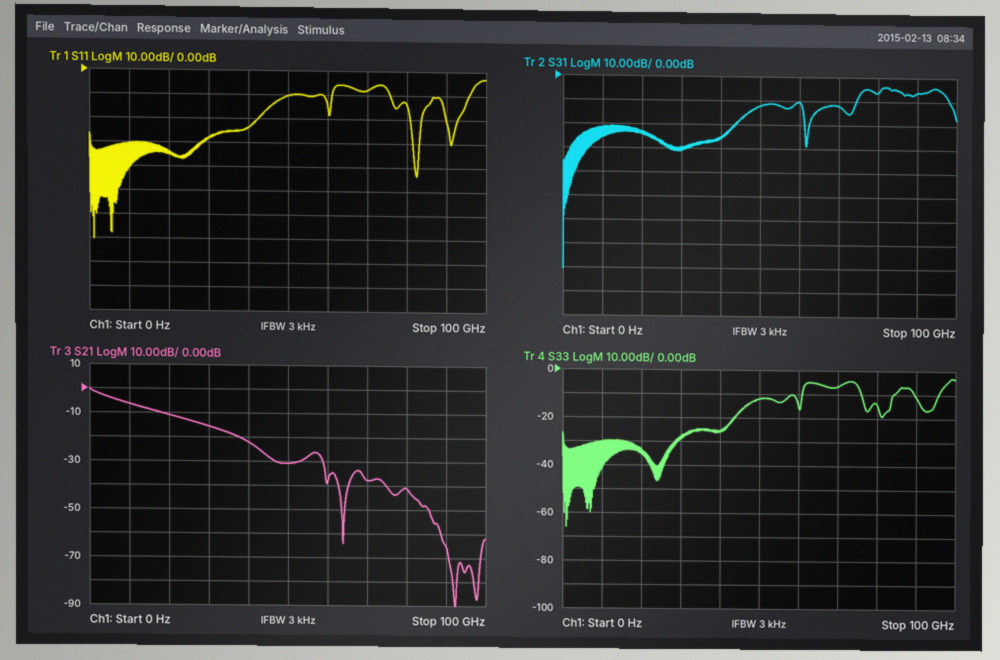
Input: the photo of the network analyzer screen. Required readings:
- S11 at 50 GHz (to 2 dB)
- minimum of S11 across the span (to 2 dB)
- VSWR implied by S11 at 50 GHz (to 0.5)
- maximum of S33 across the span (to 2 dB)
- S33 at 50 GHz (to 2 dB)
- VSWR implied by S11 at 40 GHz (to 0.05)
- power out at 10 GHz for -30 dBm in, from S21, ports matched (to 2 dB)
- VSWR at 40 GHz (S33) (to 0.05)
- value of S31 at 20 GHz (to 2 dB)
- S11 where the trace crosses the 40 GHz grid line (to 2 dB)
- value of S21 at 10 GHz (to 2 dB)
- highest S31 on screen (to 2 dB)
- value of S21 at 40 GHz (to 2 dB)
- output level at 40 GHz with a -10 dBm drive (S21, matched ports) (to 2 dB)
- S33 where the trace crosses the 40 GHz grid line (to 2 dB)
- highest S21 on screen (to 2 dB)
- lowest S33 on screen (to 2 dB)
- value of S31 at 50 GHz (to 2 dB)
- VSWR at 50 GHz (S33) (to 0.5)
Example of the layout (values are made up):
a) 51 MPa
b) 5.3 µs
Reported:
a) -10 dB
b) -70 dB
c) 2.0
d) -4 dB
e) -12 dB
f) 1.15
g) -36 dBm
h) 1.10
i) -24 dB
j) -24 dB
k) -6 dB
l) -4 dB
m) -22 dB
n) -32 dBm
o) -26 dB
p) 0 dB
q) -66 dB
r) -12 dB
s) 1.5
